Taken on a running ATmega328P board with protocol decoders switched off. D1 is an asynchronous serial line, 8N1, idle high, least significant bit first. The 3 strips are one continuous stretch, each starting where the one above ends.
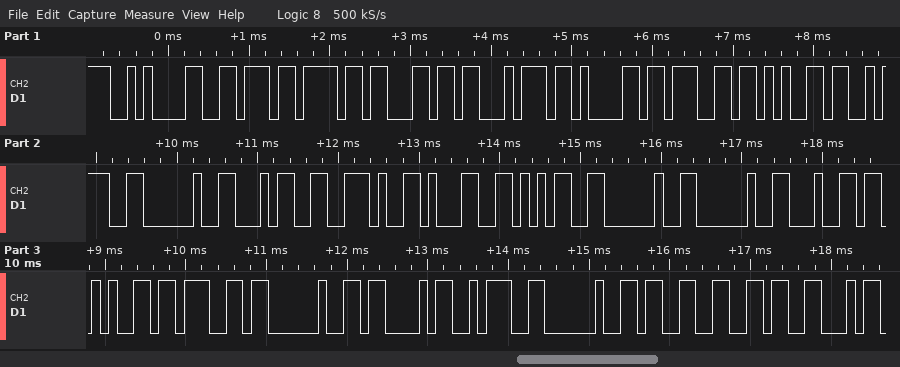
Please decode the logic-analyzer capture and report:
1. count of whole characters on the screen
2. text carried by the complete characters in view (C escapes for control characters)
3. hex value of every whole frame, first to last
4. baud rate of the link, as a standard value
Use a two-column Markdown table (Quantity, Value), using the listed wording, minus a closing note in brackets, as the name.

| Quantity | Value |
|---|---|
| count of whole characters on the screen | 25 |
| text carried by the complete characters in view | "\nvoltage: 4.15  deg C: 36" |
| hex value of every whole frame, first to last | 0A 76 6F 6C 74 61 67 65 3A 20 34 2E 31 35 20 20 64 65 67 20 43 3A 20 33 36 |
| baud rate of the link, as a standard value | 9600 baud |
